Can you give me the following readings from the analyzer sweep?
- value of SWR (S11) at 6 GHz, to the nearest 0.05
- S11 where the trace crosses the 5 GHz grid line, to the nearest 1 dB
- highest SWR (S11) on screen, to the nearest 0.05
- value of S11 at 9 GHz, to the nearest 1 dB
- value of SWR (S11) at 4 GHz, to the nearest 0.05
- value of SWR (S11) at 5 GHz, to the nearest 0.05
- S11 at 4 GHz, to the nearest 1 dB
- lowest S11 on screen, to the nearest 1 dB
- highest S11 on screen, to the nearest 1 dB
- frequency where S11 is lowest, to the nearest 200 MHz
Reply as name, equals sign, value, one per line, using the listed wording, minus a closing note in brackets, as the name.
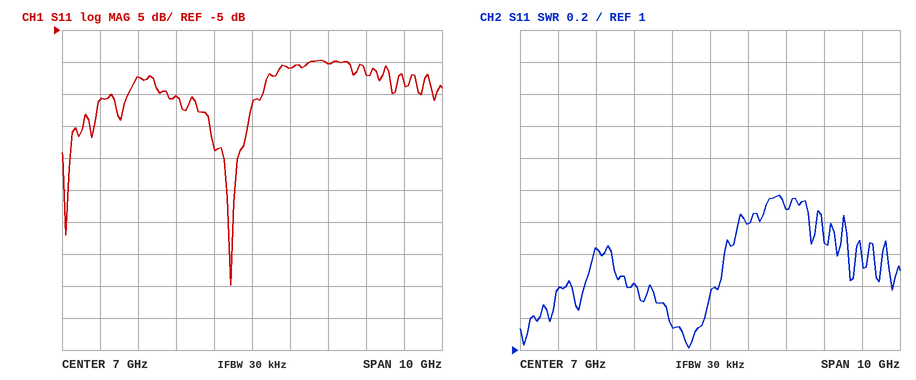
value of SWR (S11) at 6 GHz, to the nearest 0.05 = 1.15
S11 where the trace crosses the 5 GHz grid line, to the nearest 1 dB = -15 dB
highest SWR (S11) on screen, to the nearest 0.05 = 1.95
value of S11 at 9 GHz, to the nearest 1 dB = -10 dB
value of SWR (S11) at 4 GHz, to the nearest 0.05 = 1.65
value of SWR (S11) at 5 GHz, to the nearest 0.05 = 1.40
S11 at 4 GHz, to the nearest 1 dB = -12 dB
lowest S11 on screen, to the nearest 1 dB = -45 dB
highest S11 on screen, to the nearest 1 dB = -10 dB
frequency where S11 is lowest, to the nearest 200 MHz = 6.4 GHz
